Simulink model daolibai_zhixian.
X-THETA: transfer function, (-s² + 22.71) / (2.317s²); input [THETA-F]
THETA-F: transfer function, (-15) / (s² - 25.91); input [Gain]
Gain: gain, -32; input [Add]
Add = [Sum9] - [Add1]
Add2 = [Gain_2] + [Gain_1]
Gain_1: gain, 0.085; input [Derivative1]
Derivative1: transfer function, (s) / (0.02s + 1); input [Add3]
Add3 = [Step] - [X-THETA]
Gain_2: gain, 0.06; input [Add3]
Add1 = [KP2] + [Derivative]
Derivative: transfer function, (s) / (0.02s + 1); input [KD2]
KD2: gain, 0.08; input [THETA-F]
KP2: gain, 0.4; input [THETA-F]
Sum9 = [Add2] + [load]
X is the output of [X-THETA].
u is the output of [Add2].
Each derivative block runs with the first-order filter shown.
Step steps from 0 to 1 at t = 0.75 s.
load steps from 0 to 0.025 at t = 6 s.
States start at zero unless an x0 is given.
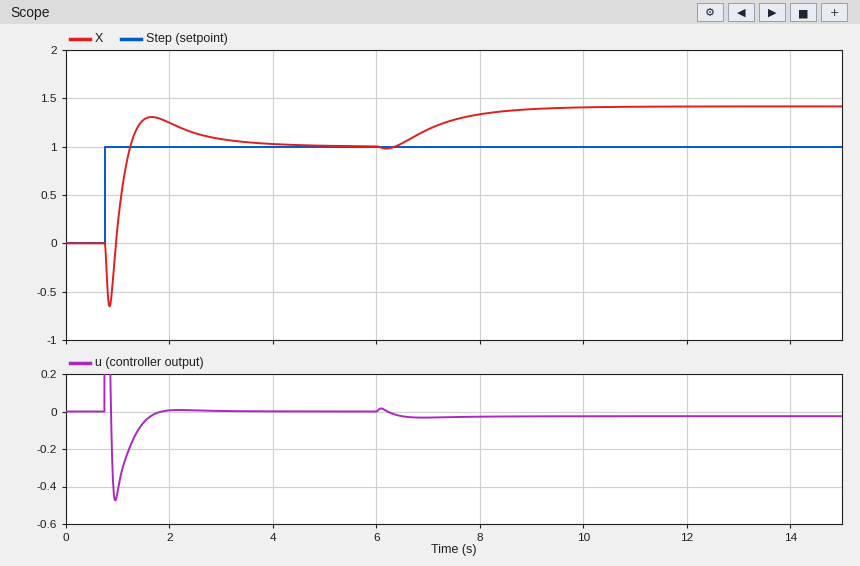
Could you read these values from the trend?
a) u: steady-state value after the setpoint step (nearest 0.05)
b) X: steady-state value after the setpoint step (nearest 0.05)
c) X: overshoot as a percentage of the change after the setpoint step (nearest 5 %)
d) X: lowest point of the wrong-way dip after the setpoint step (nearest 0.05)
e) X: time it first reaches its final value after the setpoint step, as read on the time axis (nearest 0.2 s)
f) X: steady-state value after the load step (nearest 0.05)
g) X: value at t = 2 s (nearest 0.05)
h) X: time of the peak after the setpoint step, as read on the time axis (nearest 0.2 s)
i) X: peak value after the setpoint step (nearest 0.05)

0.00
1.00
30 %
-0.65
1.2 s
1.40
1.25
1.6 s
1.30
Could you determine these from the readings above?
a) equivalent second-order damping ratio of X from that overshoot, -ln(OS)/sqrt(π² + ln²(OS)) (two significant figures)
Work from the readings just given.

0.36
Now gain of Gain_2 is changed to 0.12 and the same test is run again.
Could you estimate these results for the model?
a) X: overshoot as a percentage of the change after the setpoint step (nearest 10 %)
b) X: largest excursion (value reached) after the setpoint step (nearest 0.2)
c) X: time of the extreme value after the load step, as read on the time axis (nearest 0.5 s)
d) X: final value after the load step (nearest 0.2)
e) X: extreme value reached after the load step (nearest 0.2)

60 %
1.6
7.5 s
1.2
1.2
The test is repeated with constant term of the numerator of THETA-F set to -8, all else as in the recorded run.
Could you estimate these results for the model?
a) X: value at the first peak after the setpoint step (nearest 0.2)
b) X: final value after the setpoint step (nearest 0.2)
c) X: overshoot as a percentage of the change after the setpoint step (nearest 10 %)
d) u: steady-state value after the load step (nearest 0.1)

1.6
1.0
60 %
0.0
